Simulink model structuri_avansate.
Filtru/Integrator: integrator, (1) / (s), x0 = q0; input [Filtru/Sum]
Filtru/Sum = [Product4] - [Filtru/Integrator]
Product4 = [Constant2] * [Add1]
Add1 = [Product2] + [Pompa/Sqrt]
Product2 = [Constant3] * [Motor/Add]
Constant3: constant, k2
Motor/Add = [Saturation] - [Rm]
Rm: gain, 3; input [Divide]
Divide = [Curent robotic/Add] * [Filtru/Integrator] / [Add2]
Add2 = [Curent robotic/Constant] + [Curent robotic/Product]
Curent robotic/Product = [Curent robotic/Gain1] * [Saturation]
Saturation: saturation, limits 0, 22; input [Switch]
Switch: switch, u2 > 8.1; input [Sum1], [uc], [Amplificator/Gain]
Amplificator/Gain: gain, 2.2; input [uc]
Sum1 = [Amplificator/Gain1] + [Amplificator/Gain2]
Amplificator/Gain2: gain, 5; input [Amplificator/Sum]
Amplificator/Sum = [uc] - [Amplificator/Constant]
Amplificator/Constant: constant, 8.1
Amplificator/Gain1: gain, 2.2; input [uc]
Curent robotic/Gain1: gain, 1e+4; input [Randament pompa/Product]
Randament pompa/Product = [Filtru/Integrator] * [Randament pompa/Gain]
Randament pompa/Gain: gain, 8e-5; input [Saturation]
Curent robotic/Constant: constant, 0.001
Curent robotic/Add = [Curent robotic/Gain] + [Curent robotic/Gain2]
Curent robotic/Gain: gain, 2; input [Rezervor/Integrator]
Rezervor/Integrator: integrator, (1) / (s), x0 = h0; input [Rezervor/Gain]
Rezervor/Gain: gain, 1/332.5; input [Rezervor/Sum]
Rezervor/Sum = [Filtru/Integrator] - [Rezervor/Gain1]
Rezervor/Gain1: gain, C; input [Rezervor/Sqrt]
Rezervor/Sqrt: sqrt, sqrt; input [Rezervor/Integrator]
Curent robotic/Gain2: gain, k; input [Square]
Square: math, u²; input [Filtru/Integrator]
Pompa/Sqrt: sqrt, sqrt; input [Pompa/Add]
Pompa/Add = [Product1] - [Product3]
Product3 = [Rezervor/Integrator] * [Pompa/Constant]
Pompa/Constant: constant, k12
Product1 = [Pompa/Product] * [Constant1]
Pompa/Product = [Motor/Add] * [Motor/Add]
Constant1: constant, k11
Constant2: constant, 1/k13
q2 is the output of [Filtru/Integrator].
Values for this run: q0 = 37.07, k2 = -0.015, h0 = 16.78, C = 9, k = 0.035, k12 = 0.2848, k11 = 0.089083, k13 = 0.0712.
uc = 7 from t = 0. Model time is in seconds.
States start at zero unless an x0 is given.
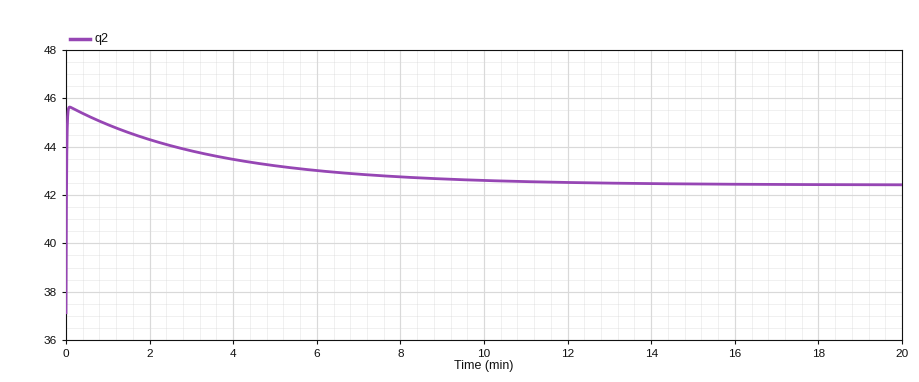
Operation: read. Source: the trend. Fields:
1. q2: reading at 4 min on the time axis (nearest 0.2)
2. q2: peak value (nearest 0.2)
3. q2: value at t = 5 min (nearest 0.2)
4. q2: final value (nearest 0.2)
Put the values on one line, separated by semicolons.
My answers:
43.4; 45.6; 43.2; 42.4
